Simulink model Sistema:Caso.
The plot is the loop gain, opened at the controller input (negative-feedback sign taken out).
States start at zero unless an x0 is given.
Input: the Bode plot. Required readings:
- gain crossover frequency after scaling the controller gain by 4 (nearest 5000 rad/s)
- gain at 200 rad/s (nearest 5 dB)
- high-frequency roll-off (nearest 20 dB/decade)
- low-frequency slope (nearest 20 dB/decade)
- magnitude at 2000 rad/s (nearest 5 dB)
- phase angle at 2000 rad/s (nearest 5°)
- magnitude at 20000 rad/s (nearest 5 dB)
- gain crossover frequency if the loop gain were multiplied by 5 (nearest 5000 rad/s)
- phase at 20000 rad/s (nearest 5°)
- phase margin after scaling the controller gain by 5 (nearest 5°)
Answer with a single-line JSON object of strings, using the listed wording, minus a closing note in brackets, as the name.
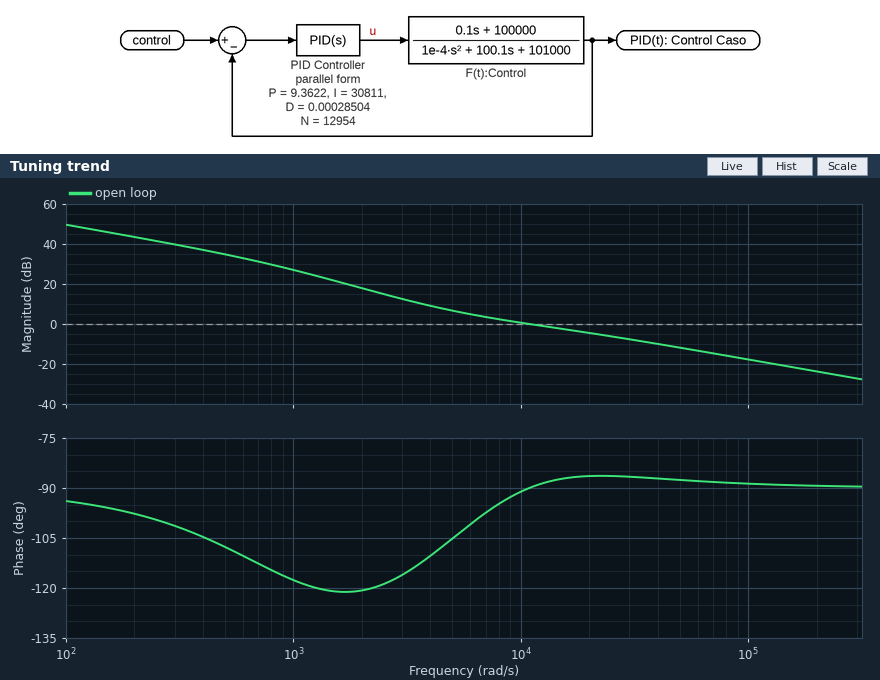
{"gain crossover frequency after scaling the controller gain by 4": "50000 rad/s", "gain at 200 rad/s": "45 dB", "high-frequency roll-off": "-20 dB/decade", "low-frequency slope": "-20 dB/decade", "magnitude at 2000 rad/s": "20 dB", "phase angle at 2000 rad/s": "-120°", "magnitude at 20000 rad/s": "-5 dB", "gain crossover frequency if the loop gain were multiplied by 5": "65000 rad/s", "phase at 20000 rad/s": "-85°", "phase margin after scaling the controller gain by 5": "90°"}
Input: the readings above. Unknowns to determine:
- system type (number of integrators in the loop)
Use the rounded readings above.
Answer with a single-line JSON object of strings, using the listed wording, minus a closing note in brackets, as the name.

{"system type": "1"}
